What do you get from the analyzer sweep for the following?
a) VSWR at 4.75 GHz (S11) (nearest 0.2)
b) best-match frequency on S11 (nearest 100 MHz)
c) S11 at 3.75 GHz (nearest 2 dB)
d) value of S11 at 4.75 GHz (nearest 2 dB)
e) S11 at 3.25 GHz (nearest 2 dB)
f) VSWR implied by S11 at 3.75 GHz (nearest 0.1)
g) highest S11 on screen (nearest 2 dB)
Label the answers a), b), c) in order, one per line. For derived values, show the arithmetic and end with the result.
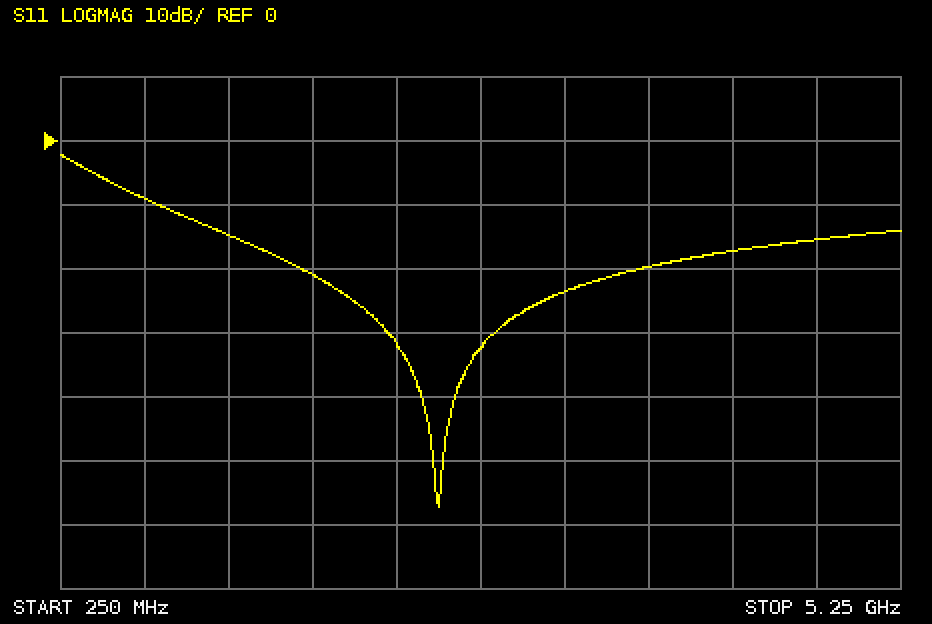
a) |Γ| = 10^(-16/20) = 0.1585; VSWR = (1 + 0.1585)/(1 − 0.1585) ≈ 1.4
b) 2.5 GHz
c) -20 dB
d) -16 dB
e) -24 dB
f) |Γ| = 10^(-20/20) = 0.1000; VSWR = (1 + 0.1000)/(1 − 0.1000) ≈ 1.2
g) -2 dB
